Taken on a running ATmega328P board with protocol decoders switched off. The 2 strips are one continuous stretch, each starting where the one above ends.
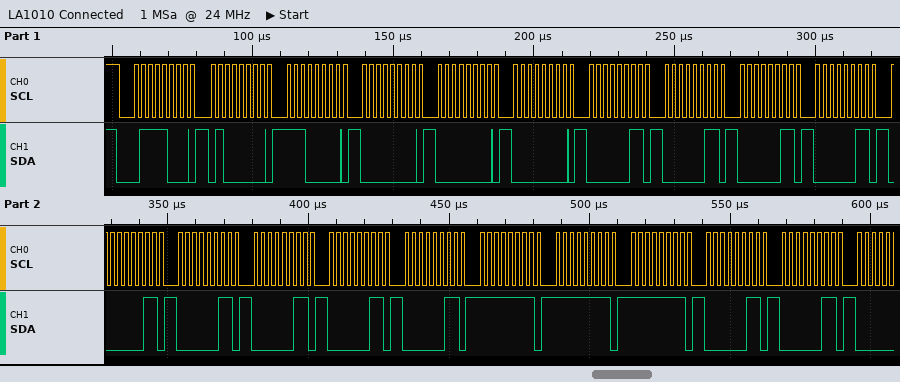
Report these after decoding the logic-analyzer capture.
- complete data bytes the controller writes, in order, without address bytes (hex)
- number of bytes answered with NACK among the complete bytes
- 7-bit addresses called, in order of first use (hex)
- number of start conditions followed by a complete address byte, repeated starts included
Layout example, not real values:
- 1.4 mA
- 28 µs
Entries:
- 40 E0 00 00 00 03 03 03 03 03 03 03 03 03 FF FF FF 03 03
- 0
- 0x3C
- 1
